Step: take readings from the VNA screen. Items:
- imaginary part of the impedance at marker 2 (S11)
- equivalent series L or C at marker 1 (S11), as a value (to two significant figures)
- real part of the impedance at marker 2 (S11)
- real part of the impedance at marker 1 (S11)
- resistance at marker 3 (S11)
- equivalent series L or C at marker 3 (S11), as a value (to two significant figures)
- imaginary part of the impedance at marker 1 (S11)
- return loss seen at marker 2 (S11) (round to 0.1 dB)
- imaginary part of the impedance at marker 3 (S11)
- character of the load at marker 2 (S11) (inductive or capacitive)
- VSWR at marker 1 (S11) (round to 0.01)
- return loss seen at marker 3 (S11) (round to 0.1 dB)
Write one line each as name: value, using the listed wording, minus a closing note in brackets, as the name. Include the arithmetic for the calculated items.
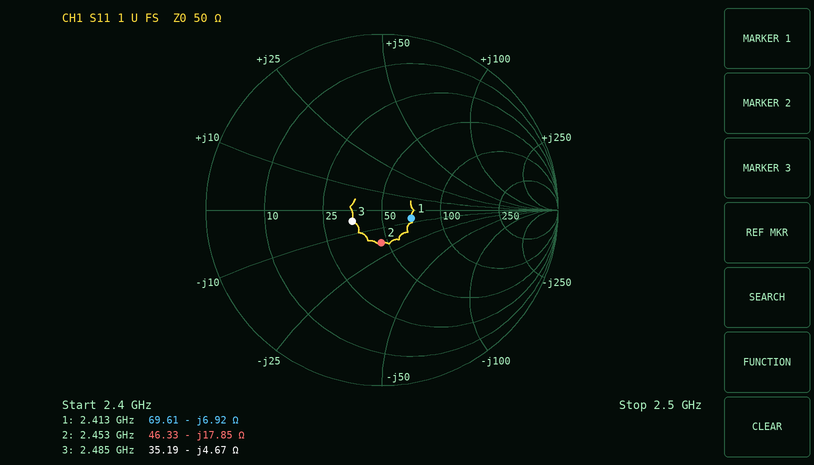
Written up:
imaginary part of the impedance at marker 2: -17.85 Ω
equivalent series L or C at marker 1 (S11), as a value: C = 1/(2π × 2.413 GHz × 6.92 Ω) ≈ 9.5 pF
real part of the impedance at marker 2: 46.33 Ω
real part of the impedance at marker 1: 69.61 Ω
resistance at marker 3: 35.19 Ω
equivalent series L or C at marker 3 (S11), as a value: C = 1/(2π × 2.485 GHz × 4.67 Ω) ≈ 14 pF
imaginary part of the impedance at marker 1: -6.92 Ω
return loss seen at marker 2 (S11): 14.6 dB
imaginary part of the impedance at marker 3: -4.67 Ω
character of the load at marker 2 (S11): capacitive
VSWR at marker 1 (S11): 1.42
return loss seen at marker 3 (S11): 14.8 dB
